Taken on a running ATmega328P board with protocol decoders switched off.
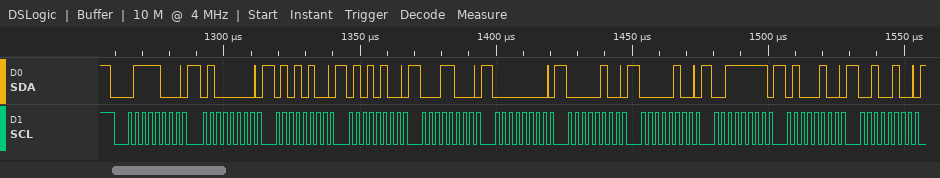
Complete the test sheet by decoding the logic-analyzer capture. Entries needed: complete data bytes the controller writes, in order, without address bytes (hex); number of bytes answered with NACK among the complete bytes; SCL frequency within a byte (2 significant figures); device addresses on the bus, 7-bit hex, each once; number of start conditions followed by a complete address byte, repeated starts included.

40 54 54 18 00 04 04 3F 44 24
0
400 kHz
0x3C
1
